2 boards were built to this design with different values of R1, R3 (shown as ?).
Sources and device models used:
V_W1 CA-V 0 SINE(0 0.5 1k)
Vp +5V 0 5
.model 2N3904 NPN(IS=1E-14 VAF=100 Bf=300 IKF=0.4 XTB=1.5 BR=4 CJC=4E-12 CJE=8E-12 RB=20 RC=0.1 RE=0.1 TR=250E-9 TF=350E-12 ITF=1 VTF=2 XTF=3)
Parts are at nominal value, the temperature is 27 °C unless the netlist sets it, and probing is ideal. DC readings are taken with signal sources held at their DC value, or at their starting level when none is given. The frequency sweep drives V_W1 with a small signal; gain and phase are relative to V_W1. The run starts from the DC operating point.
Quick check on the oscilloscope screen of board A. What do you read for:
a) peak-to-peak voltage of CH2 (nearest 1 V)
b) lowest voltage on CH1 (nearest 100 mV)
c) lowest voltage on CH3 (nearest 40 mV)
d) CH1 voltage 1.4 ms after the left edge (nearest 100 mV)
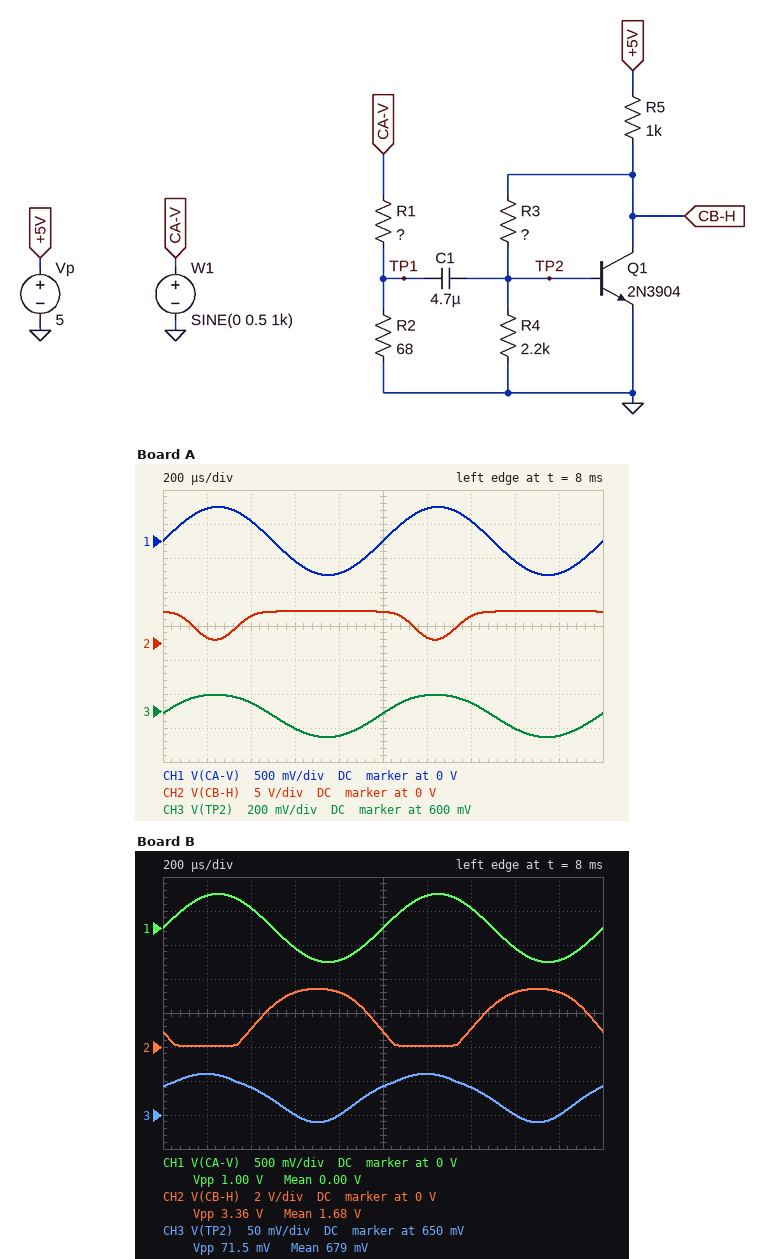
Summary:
4 V
-500 mV
440 mV
300 mV
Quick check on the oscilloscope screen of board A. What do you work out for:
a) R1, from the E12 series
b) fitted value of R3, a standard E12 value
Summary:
180 Ω
12 kΩ
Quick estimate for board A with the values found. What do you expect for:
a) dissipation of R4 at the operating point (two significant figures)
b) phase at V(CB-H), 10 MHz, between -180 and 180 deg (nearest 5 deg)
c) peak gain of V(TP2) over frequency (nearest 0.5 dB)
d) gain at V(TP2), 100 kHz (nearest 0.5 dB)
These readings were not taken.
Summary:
190 µW
160 deg
-12.0 dB
-12.0 dB
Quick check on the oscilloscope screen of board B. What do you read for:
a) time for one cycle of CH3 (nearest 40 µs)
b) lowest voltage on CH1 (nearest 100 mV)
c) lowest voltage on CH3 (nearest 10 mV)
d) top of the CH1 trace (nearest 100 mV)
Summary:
1.00 ms
-500 mV
640 mV
500 mV
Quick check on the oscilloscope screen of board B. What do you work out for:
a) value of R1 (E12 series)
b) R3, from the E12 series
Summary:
330 Ω
2.7 kΩ
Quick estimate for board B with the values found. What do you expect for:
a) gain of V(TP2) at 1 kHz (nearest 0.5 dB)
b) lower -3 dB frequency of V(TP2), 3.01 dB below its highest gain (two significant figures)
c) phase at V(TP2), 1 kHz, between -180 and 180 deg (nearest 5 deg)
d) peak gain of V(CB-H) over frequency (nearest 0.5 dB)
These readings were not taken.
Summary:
-25.0 dB
390 Hz
20 deg
14.0 dB
